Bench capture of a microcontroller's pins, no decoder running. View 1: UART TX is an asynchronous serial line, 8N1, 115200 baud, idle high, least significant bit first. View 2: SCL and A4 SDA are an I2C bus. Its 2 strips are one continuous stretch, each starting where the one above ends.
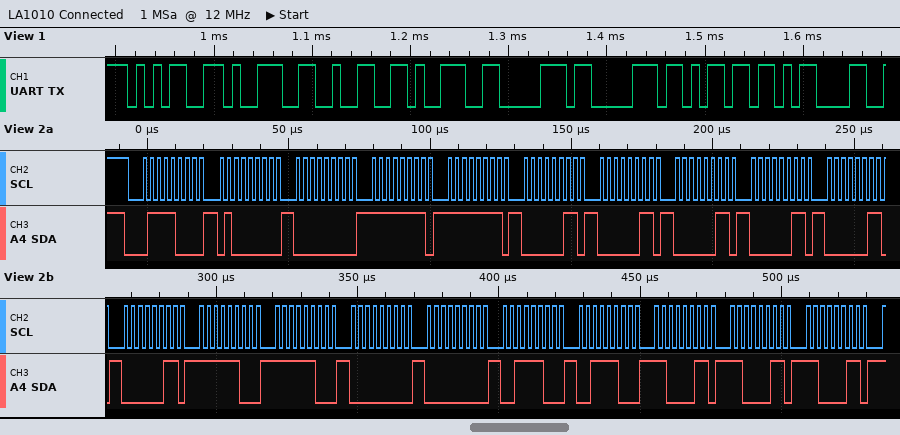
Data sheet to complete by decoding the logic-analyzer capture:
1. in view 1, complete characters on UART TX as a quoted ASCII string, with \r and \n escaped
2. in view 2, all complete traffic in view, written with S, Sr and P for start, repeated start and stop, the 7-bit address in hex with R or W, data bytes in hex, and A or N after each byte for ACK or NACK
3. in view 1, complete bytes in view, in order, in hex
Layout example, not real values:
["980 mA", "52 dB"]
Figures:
["\"5929ppm\\r\"", "S 3CW A 40 A 00 A FF A FF A 03 A 03 A 03 A 03 A 03 A 03 A FC A FC A 00 A 00 A 3C A 3C A C3 A C3 A C3 A", "0x35 0x39 0x32 0x39 0x70 0x70 0x6D 0x0D"]
